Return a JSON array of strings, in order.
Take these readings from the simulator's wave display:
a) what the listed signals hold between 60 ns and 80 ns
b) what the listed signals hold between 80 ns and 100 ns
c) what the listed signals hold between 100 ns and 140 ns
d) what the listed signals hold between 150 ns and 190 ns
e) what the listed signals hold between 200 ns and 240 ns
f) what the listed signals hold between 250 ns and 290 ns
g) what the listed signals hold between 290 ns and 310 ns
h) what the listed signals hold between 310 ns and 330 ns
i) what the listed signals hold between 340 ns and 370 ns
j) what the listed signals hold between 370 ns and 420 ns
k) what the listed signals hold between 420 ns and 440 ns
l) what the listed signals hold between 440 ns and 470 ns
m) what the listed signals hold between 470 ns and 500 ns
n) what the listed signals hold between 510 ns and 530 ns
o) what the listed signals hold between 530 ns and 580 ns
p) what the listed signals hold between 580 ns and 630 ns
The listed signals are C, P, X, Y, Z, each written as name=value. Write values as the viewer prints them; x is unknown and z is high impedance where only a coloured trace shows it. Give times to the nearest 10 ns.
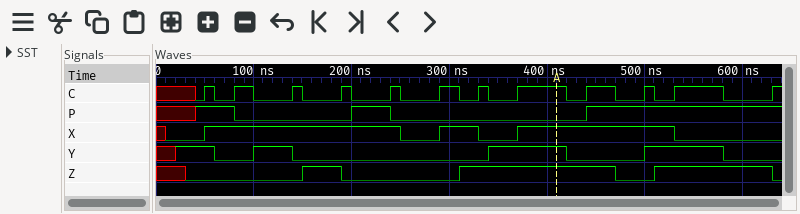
["C=0, P=1, X=1, Y=0, Z=0", "C=1, P=0, X=1, Y=0, Z=0", "C=0, P=0, X=1, Y=1, Z=0", "C=0, P=0, X=1, Y=0, Z=1", "C=0, P=1, X=1, Y=0, Z=0", "C=0, P=0, X=0, Y=0, Z=0", "C=1, P=0, X=1, Y=0, Z=0", "C=0, P=0, X=1, Y=0, Z=1", "C=0, P=0, X=0, Y=1, Z=1", "C=1, P=0, X=1, Y=1, Z=1", "C=0, P=0, X=1, Y=0, Z=1", "C=1, P=1, X=1, Y=0, Z=1", "C=0, P=1, X=1, Y=0, Z=0", "C=0, P=1, X=1, Y=1, Z=1", "C=1, P=1, X=0, Y=1, Z=1", "C=0, P=1, X=0, Y=0, Z=1"]
